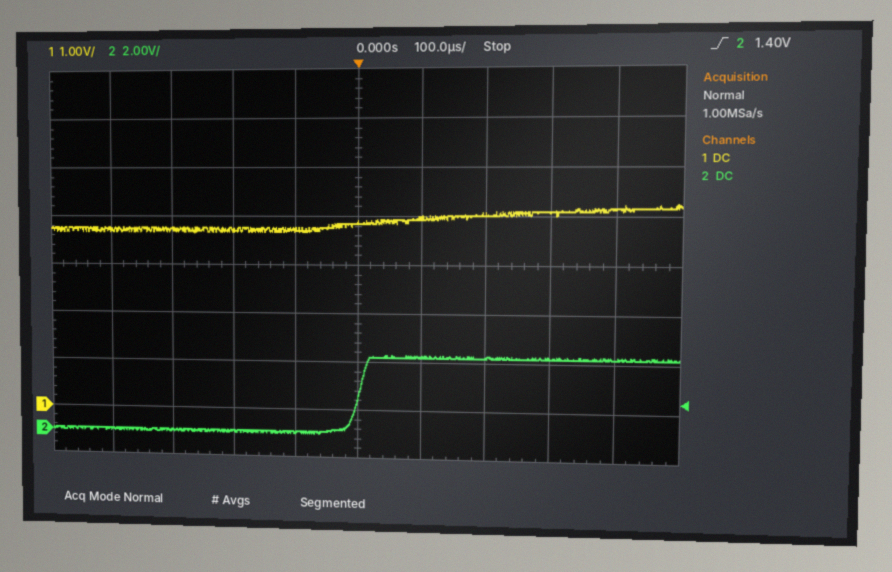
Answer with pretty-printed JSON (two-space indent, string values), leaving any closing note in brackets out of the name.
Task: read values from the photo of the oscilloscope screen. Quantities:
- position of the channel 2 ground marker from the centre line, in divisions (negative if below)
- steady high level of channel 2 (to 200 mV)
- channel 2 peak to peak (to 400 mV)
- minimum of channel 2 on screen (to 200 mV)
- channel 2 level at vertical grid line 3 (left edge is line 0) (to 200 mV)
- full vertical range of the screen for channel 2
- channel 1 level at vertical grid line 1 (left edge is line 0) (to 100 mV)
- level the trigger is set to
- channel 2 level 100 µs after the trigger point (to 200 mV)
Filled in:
{
  "position of the channel 2 ground marker from the centre line, in divisions": "-3.5 div",
  "steady high level of channel 2": "3.2 V",
  "channel 2 peak to peak": "3.2 V",
  "minimum of channel 2 on screen": "0.0 V",
  "channel 2 level at vertical grid line 3 (left edge is line 0)": "0.0 V",
  "full vertical range of the screen for channel 2": "16 V",
  "channel 1 level at vertical grid line 1 (left edge is line 0)": "3.7 V",
  "level the trigger is set to": "1.40 V",
  "channel 2 level 100 µs after the trigger point": "3.2 V"
}
